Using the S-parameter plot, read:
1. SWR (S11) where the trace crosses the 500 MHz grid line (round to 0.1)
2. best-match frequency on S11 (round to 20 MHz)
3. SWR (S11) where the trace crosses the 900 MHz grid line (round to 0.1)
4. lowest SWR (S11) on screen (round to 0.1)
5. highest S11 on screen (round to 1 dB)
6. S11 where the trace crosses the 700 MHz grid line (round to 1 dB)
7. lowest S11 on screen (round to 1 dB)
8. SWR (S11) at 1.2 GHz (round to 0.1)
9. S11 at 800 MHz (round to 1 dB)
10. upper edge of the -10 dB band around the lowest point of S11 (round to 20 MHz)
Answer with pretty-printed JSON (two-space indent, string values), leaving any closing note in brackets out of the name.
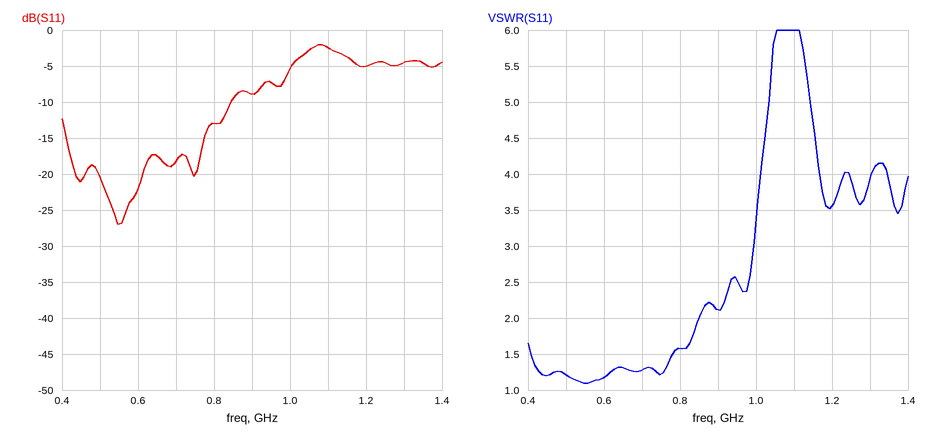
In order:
{
  "SWR (S11) where the trace crosses the 500 MHz grid line": "1.2",
  "best-match frequency on S11": "540 MHz",
  "SWR (S11) where the trace crosses the 900 MHz grid line": "2.1",
  "lowest SWR (S11) on screen": "1.1",
  "highest S11 on screen": "-2 dB",
  "S11 where the trace crosses the 700 MHz grid line": "-18 dB",
  "lowest S11 on screen": "-27 dB",
  "SWR (S11) at 1.2 GHz": "3.6",
  "S11 at 800 MHz": "-13 dB",
  "upper edge of the -10 dB band around the lowest point of S11": "840 MHz"
}
